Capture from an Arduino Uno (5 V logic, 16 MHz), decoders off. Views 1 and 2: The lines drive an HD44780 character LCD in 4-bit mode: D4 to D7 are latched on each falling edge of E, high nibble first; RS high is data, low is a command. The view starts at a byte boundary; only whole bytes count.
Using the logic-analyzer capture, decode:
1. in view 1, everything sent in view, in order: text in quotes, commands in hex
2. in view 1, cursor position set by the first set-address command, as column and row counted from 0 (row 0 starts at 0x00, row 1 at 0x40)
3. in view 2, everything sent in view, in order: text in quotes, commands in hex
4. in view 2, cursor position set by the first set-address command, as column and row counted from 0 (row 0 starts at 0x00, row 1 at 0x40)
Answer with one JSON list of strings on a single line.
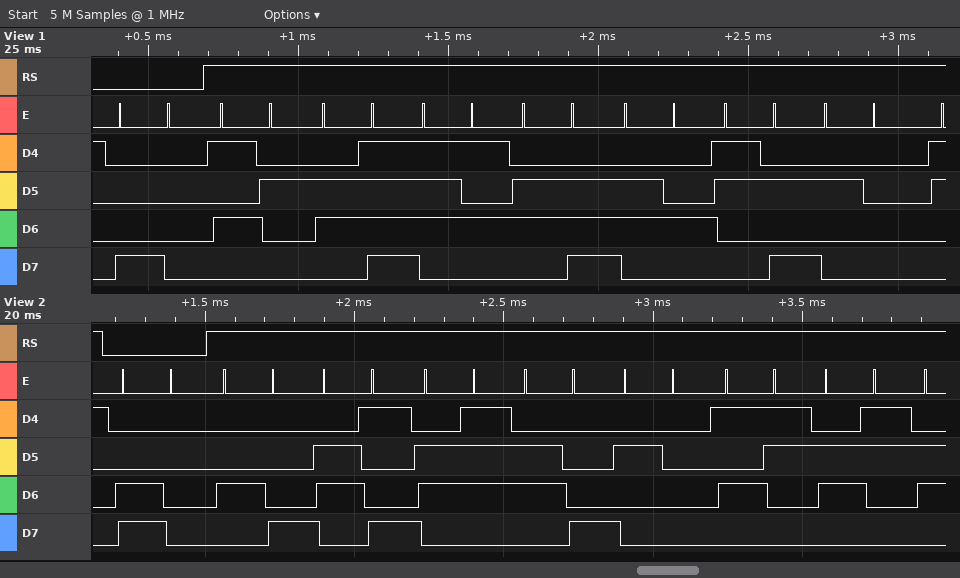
["0x80 \"Round: \"", "column 0, row 0", "0xC0 \"High Sc\"", "column 0, row 1"]
